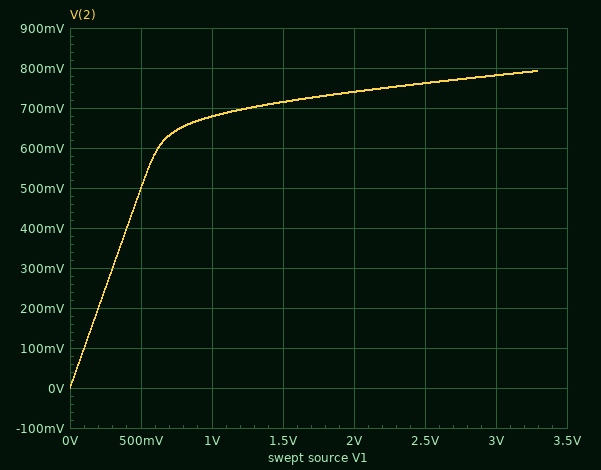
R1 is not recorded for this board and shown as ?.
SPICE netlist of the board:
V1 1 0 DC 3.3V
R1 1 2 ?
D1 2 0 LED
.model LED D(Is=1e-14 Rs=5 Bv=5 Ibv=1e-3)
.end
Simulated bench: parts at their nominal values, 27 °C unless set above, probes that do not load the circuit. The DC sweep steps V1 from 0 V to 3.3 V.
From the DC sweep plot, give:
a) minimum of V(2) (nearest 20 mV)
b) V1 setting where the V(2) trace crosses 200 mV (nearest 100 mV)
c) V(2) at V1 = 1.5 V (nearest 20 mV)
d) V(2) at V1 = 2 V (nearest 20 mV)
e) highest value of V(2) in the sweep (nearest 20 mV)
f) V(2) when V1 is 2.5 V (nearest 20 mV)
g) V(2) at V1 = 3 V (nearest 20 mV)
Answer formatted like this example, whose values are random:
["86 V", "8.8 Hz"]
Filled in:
["0 V", "200 mV", "720 mV", "740 mV", "800 mV", "760 mV", "780 mV"]
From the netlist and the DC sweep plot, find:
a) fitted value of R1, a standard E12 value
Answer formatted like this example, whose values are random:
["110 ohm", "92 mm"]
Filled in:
["180 Ω"]
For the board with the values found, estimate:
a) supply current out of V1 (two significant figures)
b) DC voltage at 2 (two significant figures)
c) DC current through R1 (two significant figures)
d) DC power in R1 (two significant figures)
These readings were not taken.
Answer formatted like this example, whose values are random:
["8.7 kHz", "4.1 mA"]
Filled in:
["14 mA", "790 mV", "14 mA", "35 mW"]
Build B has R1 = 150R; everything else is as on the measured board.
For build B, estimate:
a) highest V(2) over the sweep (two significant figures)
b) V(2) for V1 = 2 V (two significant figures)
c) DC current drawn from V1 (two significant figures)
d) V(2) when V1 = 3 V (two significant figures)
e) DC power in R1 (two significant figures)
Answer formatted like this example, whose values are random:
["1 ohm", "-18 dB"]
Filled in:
["810 mV", "750 mV", "17 mA", "800 mV", "41 mW"]
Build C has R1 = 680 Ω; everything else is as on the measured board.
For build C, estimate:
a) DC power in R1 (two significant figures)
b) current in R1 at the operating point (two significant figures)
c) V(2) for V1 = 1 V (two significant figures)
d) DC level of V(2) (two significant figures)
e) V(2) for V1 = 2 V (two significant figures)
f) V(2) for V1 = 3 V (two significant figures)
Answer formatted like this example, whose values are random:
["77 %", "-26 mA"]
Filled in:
["9.9 mW", "3.8 mA", "640 mV", "710 mV", "680 mV", "700 mV"]
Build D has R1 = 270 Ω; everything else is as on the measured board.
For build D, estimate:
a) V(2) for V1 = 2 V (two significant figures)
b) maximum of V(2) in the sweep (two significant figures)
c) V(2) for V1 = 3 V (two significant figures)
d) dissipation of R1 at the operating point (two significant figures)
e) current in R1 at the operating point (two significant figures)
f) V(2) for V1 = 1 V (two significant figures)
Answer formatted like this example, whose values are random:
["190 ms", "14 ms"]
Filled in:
["720 mV", "760 mV", "750 mV", "24 mW", "9.4 mA", "670 mV"]
